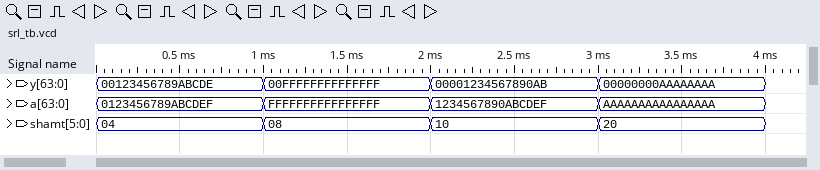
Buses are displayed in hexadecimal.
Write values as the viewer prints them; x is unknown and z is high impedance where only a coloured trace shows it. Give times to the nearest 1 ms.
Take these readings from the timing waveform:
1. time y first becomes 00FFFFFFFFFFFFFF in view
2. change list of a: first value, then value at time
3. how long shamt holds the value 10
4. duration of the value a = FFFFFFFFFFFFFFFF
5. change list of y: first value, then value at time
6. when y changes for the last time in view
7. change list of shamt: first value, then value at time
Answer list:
1 ms
0123456789ABCDEF, FFFFFFFFFFFFFFFF at 1 ms, 1234567890ABCDEF at 2 ms, AAAAAAAAAAAAAAAA at 3 ms
1 ms
1 ms
00123456789ABCDE, 00FFFFFFFFFFFFFF at 1 ms, 00001234567890AB at 2 ms, 00000000AAAAAAAA at 3 ms
3 ms
04, 08 at 1 ms, 10 at 2 ms, 20 at 3 ms
